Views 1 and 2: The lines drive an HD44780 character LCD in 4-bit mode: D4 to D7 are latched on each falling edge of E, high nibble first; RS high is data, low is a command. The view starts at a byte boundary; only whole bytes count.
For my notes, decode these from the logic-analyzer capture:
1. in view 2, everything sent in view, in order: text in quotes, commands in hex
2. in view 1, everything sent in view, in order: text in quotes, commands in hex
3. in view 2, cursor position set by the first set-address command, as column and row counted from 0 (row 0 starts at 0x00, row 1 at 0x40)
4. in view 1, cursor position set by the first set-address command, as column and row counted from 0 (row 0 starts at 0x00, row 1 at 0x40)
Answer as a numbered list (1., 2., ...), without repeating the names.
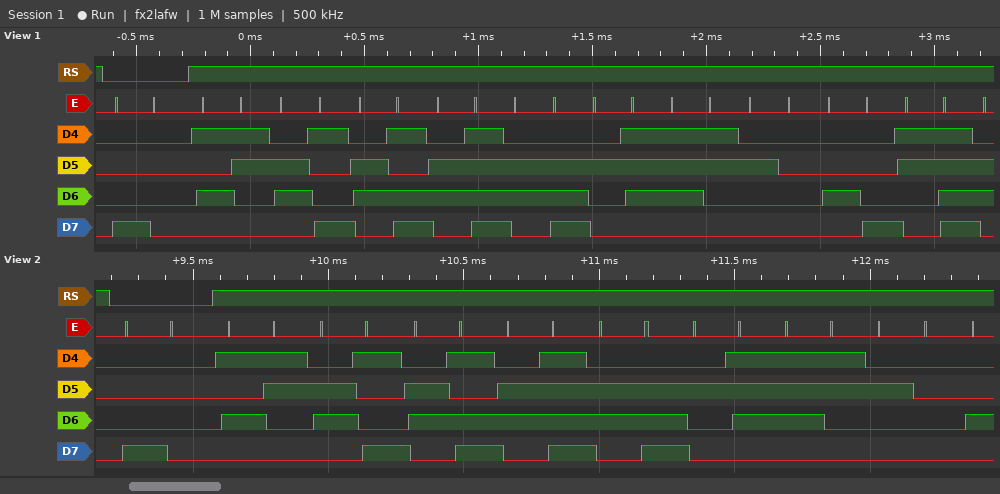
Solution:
1. 0x80 "Simon's "
2. 0x80 "Simon's H?"
3. column 0, row 0
4. column 0, row 0
